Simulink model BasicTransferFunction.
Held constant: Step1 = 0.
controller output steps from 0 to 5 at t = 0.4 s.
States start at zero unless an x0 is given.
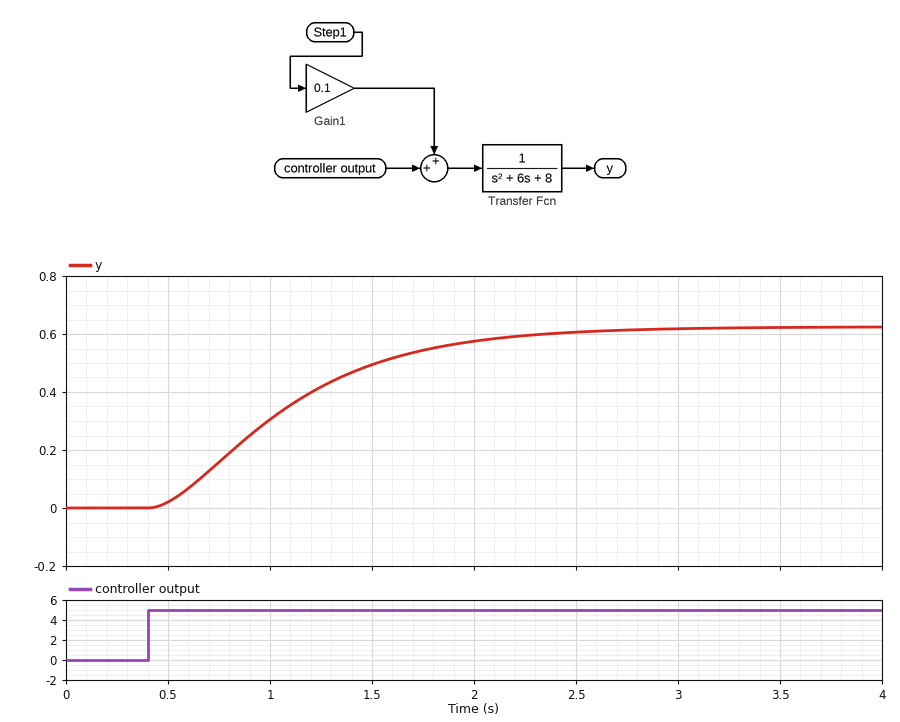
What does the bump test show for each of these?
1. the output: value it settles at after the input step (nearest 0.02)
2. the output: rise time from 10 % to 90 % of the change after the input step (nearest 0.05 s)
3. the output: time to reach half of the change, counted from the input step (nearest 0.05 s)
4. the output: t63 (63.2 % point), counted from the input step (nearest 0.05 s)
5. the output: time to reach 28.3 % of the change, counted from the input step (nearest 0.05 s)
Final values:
0.62
1.30 s
0.60 s
0.80 s
0.40 s
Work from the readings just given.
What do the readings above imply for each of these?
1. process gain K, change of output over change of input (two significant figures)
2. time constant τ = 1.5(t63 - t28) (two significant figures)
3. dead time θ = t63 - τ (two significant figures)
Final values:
0.12
0.60 s
0.20 s
